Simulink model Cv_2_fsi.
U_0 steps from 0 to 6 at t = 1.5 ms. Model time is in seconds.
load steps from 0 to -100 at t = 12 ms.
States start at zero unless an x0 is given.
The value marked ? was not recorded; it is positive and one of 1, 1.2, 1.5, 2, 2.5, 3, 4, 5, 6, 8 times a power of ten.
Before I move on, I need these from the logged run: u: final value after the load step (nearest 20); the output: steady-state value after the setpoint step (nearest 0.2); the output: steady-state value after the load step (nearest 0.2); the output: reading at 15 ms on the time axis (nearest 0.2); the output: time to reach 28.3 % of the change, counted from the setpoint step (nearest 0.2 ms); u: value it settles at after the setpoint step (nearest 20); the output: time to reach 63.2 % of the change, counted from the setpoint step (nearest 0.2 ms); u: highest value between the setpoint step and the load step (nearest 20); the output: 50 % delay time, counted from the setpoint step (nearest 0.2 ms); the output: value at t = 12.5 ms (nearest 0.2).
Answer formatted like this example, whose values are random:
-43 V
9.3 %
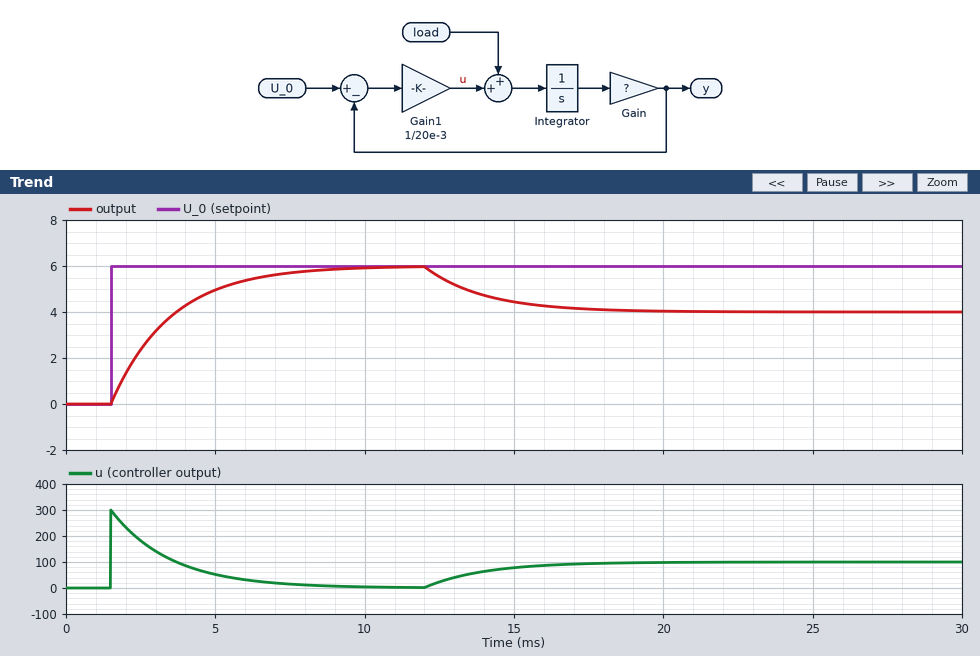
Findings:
100
6.0
4.0
4.4
0.6 ms
0
2.0 ms
300
1.4 ms
5.6
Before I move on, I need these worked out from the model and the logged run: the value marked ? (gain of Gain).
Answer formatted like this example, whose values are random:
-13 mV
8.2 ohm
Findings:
10
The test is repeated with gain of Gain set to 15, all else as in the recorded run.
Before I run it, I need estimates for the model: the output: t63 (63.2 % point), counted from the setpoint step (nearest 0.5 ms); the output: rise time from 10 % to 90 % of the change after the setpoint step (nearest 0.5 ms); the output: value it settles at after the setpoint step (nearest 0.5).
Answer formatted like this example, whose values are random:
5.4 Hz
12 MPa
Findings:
1.5 ms
3.0 ms
6.0
